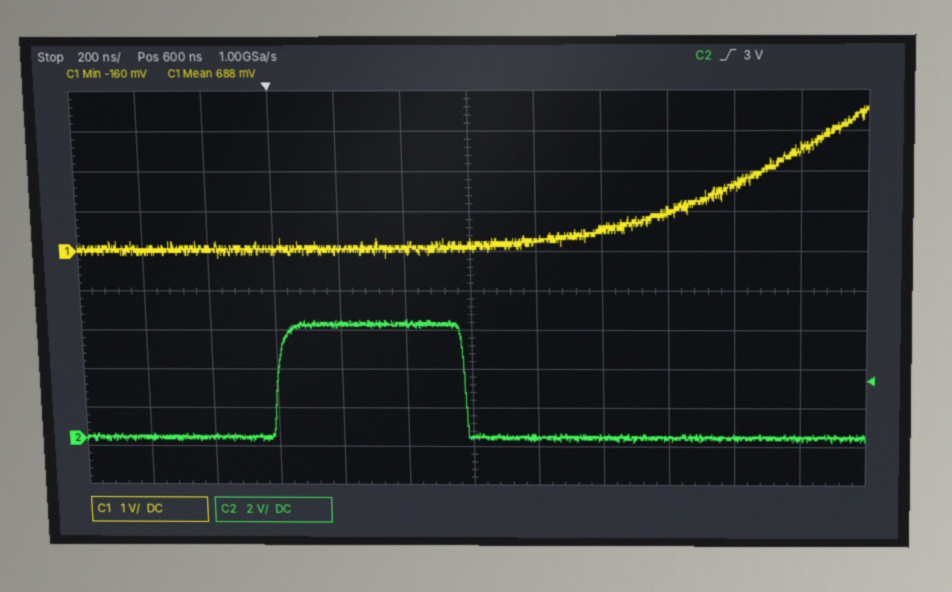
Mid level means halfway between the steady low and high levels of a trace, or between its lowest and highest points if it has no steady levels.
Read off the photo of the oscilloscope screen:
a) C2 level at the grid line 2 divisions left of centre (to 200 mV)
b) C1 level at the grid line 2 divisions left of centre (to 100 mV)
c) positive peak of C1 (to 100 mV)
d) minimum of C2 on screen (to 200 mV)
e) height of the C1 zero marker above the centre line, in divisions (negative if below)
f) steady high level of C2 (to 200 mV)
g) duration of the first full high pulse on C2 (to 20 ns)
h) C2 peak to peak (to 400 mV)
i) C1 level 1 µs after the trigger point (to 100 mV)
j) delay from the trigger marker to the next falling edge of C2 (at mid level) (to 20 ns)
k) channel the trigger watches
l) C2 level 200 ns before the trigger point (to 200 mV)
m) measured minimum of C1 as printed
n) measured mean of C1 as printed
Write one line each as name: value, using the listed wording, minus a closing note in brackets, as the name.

C2 level at the grid line 2 divisions left of centre: 6.0 V
C1 level at the grid line 2 divisions left of centre: 100 mV
positive peak of C1: 3.6 V
minimum of C2 on screen: -200 mV
height of the C1 zero marker above the centre line, in divisions: +1.0 div
steady high level of C2: 6.0 V
duration of the first full high pulse on C2: 580 ns
C2 peak to peak: 6.4 V
C1 level 1 µs after the trigger point: 600 mV
delay from the trigger marker to the next falling edge of C2 (at mid level): 580 ns
channel the trigger watches: C2
C2 level 200 ns before the trigger point: 200 mV
measured minimum of C1 as printed: -160 mV
measured mean of C1 as printed: 688 mV
